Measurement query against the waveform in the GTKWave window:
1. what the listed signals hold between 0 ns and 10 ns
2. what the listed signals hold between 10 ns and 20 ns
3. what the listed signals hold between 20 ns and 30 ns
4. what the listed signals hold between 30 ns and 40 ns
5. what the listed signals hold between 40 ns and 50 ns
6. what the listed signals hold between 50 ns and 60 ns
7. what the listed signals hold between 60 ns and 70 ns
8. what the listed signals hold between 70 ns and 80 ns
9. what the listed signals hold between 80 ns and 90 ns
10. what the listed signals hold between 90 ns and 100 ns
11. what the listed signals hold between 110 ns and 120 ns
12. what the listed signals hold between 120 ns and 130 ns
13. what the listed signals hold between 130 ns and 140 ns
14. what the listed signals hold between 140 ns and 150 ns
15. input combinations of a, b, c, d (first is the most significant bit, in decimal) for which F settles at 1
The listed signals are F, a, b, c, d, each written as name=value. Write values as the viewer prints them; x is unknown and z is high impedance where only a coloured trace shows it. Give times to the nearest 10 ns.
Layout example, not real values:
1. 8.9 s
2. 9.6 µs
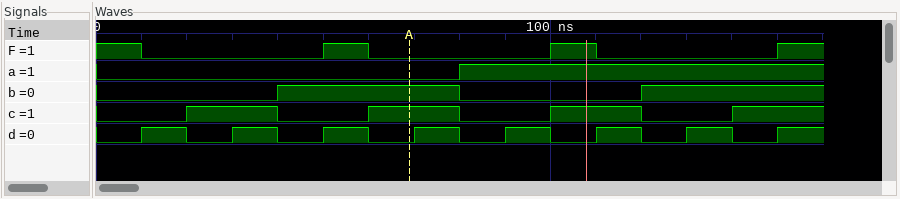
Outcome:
1. F=1, a=0, b=0, c=0, d=0
2. F=0, a=0, b=0, c=0, d=1
3. F=0, a=0, b=0, c=1, d=0
4. F=0, a=0, b=0, c=1, d=1
5. F=0, a=0, b=1, c=0, d=0
6. F=1, a=0, b=1, c=0, d=1
7. F=0, a=0, b=1, c=1, d=0
8. F=0, a=0, b=1, c=1, d=1
9. F=0, a=1, b=0, c=0, d=0
10. F=0, a=1, b=0, c=0, d=1
11. F=0, a=1, b=0, c=1, d=1
12. F=0, a=1, b=1, c=0, d=0
13. F=0, a=1, b=1, c=0, d=1
14. F=0, a=1, b=1, c=1, d=0
15. 0, 5, 10, 15
